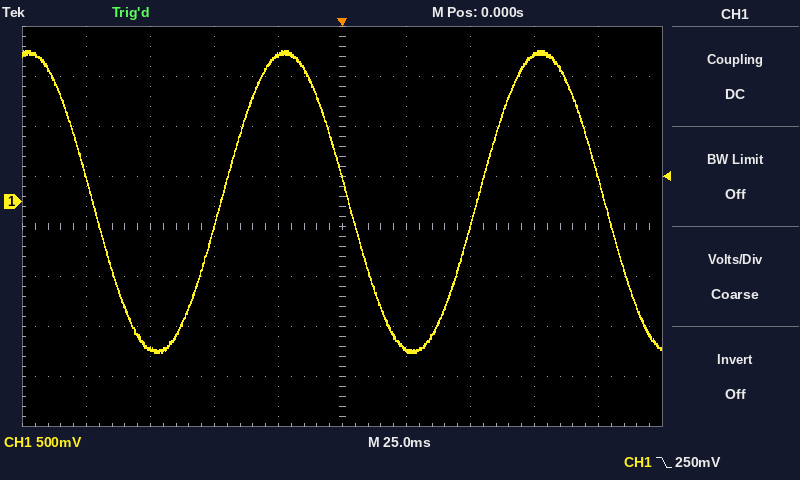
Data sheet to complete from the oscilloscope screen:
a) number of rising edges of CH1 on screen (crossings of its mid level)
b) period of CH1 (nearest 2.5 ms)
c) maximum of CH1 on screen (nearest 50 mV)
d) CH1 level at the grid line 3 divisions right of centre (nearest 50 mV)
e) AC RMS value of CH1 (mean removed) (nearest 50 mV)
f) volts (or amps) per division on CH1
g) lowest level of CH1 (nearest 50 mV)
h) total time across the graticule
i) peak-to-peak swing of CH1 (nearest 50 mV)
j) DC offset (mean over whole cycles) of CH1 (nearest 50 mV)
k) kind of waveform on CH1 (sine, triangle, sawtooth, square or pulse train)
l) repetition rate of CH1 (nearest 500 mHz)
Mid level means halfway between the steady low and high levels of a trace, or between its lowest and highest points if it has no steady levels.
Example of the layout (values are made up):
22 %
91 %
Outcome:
2
100.0 ms
1.50 V
1.45 V
1.05 V
500 mV
-1.50 V
250 ms
3.00 V
0 mV
sine
10.0 Hz
